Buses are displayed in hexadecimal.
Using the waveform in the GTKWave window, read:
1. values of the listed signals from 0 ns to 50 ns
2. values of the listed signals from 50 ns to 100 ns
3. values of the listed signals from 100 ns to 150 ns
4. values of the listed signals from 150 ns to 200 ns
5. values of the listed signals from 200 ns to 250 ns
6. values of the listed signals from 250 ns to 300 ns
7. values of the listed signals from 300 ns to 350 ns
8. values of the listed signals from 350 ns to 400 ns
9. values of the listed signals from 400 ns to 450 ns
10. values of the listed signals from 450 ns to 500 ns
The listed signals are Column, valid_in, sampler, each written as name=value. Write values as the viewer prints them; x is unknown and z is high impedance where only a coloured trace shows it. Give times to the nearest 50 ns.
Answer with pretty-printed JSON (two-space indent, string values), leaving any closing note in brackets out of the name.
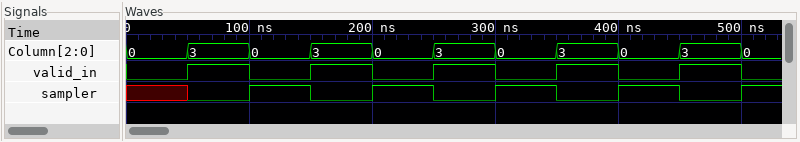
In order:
{
  "values of the listed signals from 0 ns to 50 ns": "Column=0, valid_in=0, sampler=x",
  "values of the listed signals from 50 ns to 100 ns": "Column=3, valid_in=1, sampler=0",
  "values of the listed signals from 100 ns to 150 ns": "Column=0, valid_in=0, sampler=1",
  "values of the listed signals from 150 ns to 200 ns": "Column=3, valid_in=1, sampler=0",
  "values of the listed signals from 200 ns to 250 ns": "Column=0, valid_in=0, sampler=1",
  "values of the listed signals from 250 ns to 300 ns": "Column=3, valid_in=1, sampler=0",
  "values of the listed signals from 300 ns to 350 ns": "Column=0, valid_in=0, sampler=1",
  "values of the listed signals from 350 ns to 400 ns": "Column=3, valid_in=1, sampler=0",
  "values of the listed signals from 400 ns to 450 ns": "Column=0, valid_in=0, sampler=1",
  "values of the listed signals from 450 ns to 500 ns": "Column=3, valid_in=1, sampler=0"
}
